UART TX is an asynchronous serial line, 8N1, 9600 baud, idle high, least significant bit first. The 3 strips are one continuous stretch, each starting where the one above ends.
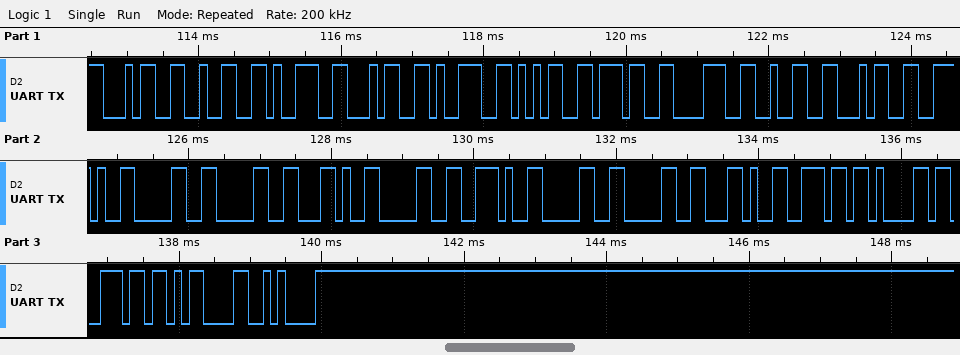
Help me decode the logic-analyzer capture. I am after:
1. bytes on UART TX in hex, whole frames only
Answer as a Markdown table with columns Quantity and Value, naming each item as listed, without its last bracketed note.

| Quantity | Value |
|---|---|
| bytes on UART TX in hex, whole frames only | 34 32 39 34 39 35 37 38 32 34 2E 30 30 2C 30 2E 30 30 2C 6E 61 6E 0D 0A |
